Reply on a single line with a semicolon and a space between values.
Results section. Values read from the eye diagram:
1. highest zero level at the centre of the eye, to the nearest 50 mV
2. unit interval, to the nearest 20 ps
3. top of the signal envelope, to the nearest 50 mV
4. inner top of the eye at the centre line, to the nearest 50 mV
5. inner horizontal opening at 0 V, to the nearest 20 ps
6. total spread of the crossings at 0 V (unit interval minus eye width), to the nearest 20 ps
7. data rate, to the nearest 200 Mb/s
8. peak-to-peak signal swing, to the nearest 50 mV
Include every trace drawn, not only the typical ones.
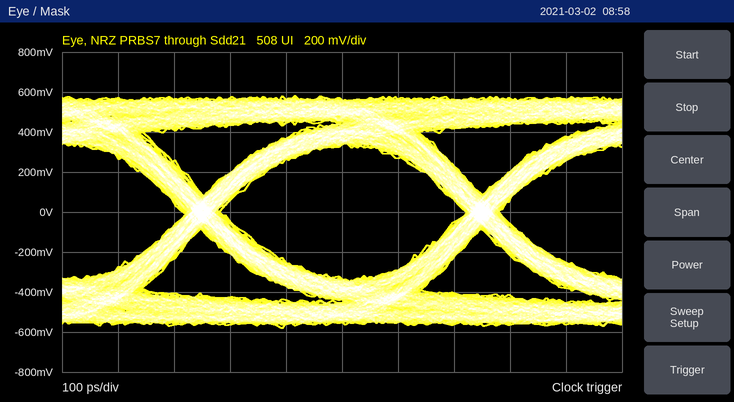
-350 mV; 500 ps; 600 mV; 350 mV; 440 ps; 60 ps; 2.0 Gb/s; 1.15 V
